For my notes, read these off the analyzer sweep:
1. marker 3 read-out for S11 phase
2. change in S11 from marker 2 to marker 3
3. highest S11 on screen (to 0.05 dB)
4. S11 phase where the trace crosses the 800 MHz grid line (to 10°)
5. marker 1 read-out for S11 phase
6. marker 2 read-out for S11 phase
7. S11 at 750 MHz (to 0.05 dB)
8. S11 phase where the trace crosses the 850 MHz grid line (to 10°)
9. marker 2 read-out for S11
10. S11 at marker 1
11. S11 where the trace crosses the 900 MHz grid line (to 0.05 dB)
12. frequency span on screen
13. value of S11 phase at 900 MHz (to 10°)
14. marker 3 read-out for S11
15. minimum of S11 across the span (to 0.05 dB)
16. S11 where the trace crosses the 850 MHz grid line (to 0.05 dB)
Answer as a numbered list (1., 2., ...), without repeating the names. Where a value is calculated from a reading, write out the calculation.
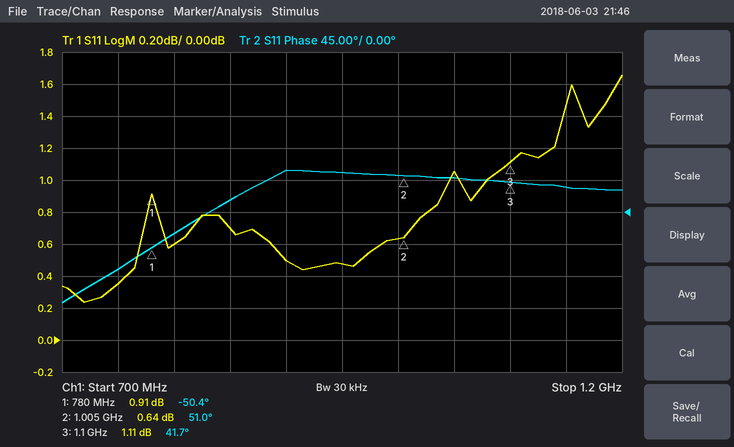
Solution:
1. 41.7°
2. 1.11 − (0.64) = 0.47 dB
3. 1.65 dB
4. -30°
5. -50.4°
6. 51.0°
7. 0.35 dB
8. 20°
9. 0.64 dB
10. 0.91 dB
11. 0.50 dB
12. 500 MHz
13. 60°
14. 1.11 dB
15. 0.25 dB
16. 0.70 dB
